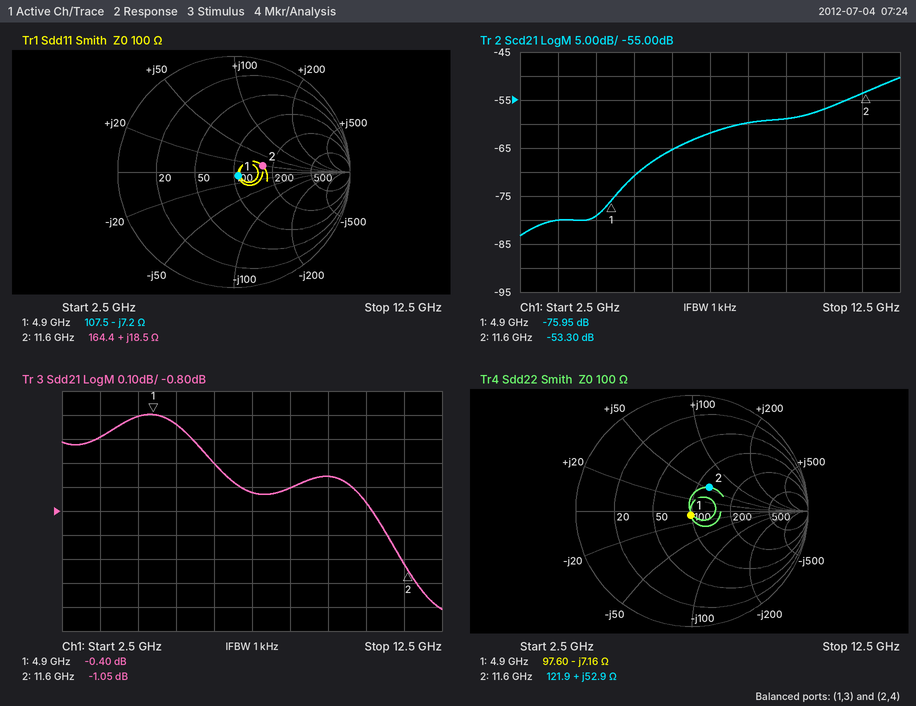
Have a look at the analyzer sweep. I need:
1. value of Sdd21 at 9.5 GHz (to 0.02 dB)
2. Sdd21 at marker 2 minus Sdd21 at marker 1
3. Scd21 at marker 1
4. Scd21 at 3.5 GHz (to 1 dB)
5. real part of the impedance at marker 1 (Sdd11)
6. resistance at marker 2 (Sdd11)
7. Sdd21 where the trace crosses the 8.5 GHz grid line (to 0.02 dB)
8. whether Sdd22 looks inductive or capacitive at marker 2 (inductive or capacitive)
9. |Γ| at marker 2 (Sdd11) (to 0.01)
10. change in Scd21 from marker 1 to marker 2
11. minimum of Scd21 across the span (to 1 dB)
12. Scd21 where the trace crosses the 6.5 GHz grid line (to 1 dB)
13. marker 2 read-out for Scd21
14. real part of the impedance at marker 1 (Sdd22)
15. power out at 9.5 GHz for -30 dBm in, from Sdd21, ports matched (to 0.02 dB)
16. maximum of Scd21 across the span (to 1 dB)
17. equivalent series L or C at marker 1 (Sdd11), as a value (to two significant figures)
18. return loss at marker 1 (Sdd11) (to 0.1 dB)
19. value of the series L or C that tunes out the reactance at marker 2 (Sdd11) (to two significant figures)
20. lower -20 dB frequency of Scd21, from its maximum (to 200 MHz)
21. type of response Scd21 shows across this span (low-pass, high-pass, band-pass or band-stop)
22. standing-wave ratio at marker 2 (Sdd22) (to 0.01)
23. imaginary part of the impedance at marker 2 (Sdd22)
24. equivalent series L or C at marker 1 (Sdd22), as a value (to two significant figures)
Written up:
-0.66 dB
-0.65 dB
-75.95 dB
-80 dB
107.5 Ω
164.4 Ω
-0.70 dB
inductive
0.25
22.65 dB
-83 dB
-65 dB
-53.30 dB
97.60 Ω
-30.66 dBm
-50 dB
4.5 pF
26.0 dB
740 fF
5.6 GHz
high-pass
1.67
+52.9 Ω
4.5 pF
